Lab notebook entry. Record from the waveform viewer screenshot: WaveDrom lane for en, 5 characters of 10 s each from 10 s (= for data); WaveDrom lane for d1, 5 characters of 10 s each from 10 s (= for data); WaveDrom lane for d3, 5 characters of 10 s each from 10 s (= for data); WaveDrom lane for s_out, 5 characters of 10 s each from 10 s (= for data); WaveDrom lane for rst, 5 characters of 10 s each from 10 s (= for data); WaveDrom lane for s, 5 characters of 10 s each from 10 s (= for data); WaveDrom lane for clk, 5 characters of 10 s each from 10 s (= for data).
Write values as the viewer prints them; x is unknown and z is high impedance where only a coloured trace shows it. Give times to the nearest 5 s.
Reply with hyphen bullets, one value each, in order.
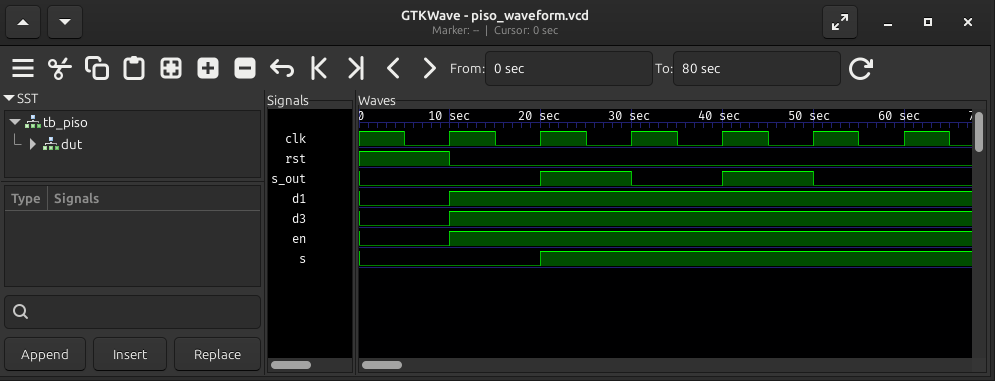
- {name: 'en', wave: '1....'}
- {name: 'd1', wave: '1....'}
- {name: 'd3', wave: '1....'}
- {name: 's_out', wave: '01010'}
- {name: 'rst', wave: '0....'}
- {name: 's', wave: '01...'}
- {name: 'clk', wave: 'p....'}
